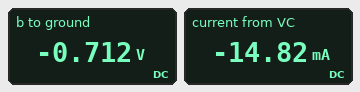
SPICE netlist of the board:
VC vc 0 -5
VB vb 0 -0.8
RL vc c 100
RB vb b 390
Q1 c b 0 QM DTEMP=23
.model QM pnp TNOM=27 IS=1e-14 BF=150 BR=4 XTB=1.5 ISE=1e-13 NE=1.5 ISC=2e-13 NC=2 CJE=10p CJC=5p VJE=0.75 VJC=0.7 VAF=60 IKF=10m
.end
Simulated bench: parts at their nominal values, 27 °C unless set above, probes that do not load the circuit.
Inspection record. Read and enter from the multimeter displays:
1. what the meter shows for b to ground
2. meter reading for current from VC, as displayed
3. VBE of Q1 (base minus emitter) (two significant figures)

-0.712 V
-14.82 mA
-710 mV
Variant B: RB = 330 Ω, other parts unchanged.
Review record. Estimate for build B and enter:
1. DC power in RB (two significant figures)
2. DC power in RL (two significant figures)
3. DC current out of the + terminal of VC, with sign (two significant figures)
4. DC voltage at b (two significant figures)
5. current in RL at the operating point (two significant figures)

21 µW
26 mW
-16 mA
-720 mV
16 mA
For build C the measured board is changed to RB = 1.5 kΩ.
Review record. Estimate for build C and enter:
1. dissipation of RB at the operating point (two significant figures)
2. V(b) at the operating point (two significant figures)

9.3 µW
-680 mV
